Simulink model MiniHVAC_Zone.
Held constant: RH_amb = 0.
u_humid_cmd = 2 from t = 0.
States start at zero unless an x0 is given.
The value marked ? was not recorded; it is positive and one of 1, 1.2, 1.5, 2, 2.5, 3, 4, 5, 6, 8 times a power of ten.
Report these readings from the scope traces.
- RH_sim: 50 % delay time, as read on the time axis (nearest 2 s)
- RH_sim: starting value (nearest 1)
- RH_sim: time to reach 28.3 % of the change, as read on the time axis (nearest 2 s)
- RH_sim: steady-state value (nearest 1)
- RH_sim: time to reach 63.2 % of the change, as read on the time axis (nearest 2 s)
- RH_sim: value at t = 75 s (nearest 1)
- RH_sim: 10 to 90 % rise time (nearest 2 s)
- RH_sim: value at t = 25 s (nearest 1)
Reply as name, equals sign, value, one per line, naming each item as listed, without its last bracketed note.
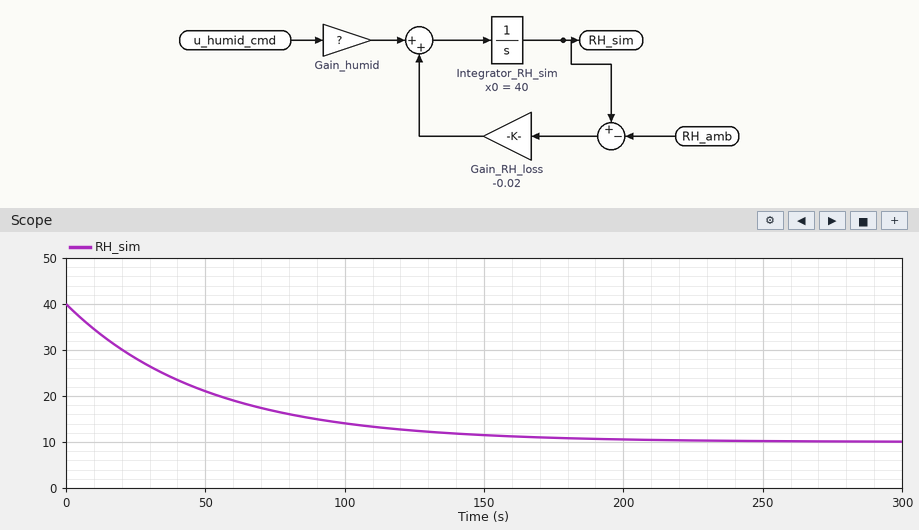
RH_sim: 50 % delay time, as read on the time axis = 34 s
RH_sim: starting value = 40
RH_sim: time to reach 28.3 % of the change, as read on the time axis = 16 s
RH_sim: steady-state value = 10
RH_sim: time to reach 63.2 % of the change, as read on the time axis = 50 s
RH_sim: value at t = 75 s = 17
RH_sim: 10 to 90 % rise time = 110 s
RH_sim: value at t = 25 s = 28
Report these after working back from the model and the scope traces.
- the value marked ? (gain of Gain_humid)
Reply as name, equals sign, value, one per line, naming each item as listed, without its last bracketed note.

the value marked ? = 0.1
